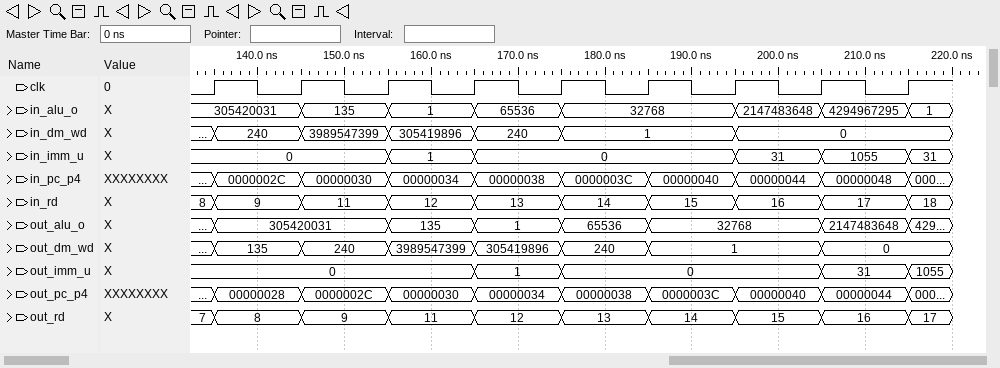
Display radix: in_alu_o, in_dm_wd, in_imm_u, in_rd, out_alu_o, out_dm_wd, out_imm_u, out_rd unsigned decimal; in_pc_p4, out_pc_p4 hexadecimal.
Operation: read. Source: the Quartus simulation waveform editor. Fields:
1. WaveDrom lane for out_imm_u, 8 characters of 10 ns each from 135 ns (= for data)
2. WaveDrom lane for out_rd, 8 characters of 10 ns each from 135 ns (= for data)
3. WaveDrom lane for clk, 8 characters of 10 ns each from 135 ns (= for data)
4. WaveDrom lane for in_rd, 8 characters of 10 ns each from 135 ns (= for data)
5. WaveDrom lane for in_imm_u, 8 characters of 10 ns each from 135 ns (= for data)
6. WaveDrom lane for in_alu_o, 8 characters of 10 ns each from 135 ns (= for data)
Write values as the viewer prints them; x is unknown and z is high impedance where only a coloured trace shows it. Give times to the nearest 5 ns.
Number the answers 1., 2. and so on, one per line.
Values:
1. {name: 'out_imm_u', wave: '=..==..=', data: '0 1 0 31'}
2. {name: 'out_rd', wave: '========', data: '8 9 11 12 13 14 15 16'}
3. {name: 'clk', wave: 'p.......'}
4. {name: 'in_rd', wave: '========', data: '9 11 12 13 14 15 16 17'}
5. {name: 'in_imm_u', wave: '=.==..==', data: '0 1 0 31 1055'}
6. {name: 'in_alu_o', wave: '=====.==', data: '305420031 135 1 65536 32768 2147483648 4294967295'}
